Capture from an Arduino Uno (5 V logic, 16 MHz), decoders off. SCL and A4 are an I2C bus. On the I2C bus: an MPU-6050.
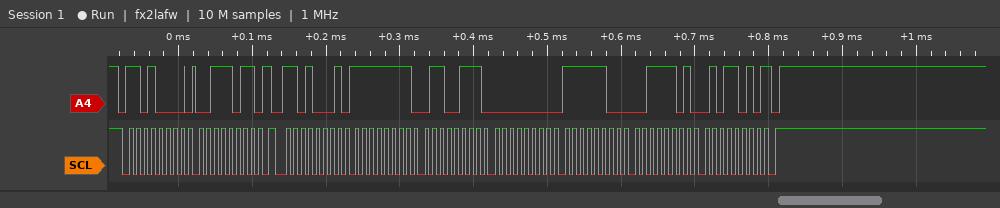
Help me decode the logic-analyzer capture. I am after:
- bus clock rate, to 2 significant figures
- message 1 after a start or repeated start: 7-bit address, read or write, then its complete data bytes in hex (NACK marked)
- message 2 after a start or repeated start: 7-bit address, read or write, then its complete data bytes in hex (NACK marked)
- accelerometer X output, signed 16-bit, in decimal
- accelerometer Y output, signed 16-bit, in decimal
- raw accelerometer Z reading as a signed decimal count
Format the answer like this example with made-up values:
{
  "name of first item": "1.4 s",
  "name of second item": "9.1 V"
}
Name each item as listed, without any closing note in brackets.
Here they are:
{
  "bus clock rate, to 2 significant figures": "100 kHz",
  "message 1 after a start or repeated start: 7-bit address, read or write, then its complete data bytes in hex": "0x68 write: 3B",
  "message 2 after a start or repeated start: 7-bit address, read or write, then its complete data bytes in hex": "0x68 read: FF 67 00 FC 3D 5A NACK",
  "accelerometer X output, signed 16-bit, in decimal": "-153",
  "accelerometer Y output, signed 16-bit, in decimal": "252",
  "raw accelerometer Z reading as a signed decimal count": "15706"
}
